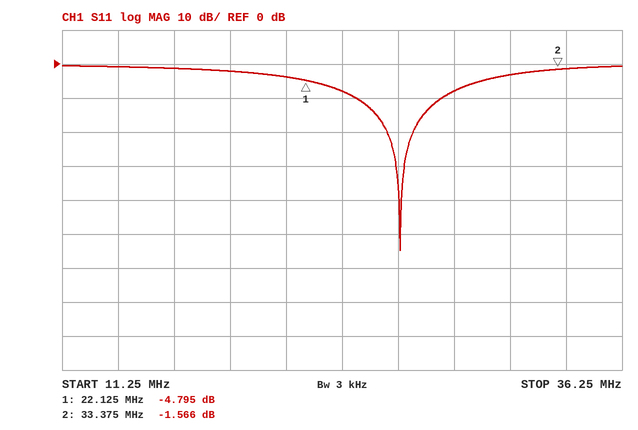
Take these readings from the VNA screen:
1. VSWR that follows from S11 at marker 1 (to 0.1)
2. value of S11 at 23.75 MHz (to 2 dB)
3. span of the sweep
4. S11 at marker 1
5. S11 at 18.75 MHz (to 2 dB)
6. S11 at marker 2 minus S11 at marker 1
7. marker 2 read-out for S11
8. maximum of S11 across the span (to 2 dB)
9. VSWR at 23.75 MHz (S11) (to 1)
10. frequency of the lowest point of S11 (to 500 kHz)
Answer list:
3.7
-8 dB
25 MHz
-4.795 dB
-2 dB
3.229 dB
-1.566 dB
0 dB
2
26.5 MHz
